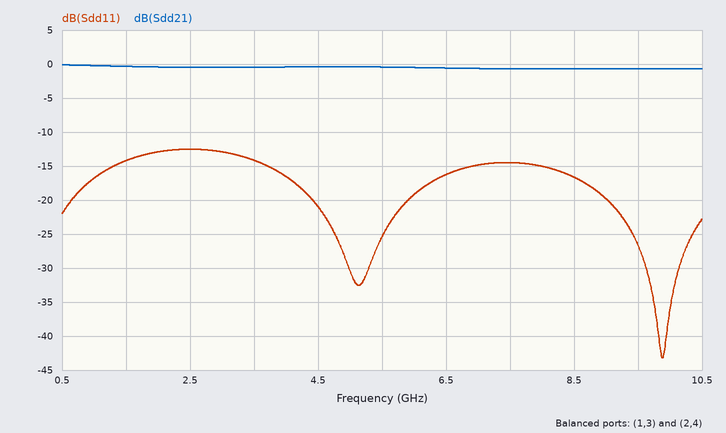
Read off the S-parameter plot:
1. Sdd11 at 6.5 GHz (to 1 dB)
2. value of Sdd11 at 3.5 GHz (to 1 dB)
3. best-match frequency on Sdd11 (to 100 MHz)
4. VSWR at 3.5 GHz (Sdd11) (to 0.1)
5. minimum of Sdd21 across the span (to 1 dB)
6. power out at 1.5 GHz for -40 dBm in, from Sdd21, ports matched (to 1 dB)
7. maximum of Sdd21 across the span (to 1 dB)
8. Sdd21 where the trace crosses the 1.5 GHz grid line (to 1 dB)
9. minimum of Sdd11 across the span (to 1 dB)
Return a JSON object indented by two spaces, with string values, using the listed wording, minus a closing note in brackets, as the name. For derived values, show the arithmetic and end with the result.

{
  "Sdd11 at 6.5 GHz": "-16 dB",
  "value of Sdd11 at 3.5 GHz": "-14 dB",
  "best-match frequency on Sdd11": "9.9 GHz",
  "VSWR at 3.5 GHz (Sdd11)": "|Γ| = 10^(-14/20) = 0.1995; VSWR = (1 + 0.1995)/(1 − 0.1995) ≈ 1.5",
  "minimum of Sdd21 across the span": "-1 dB",
  "power out at 1.5 GHz for -40 dBm in, from Sdd21, ports matched": "-40 dBm + (0 dB) = -40 dBm",
  "maximum of Sdd21 across the span": "0 dB",
  "Sdd21 where the trace crosses the 1.5 GHz grid line": "0 dB",
  "minimum of Sdd11 across the span": "-43 dB"
}
